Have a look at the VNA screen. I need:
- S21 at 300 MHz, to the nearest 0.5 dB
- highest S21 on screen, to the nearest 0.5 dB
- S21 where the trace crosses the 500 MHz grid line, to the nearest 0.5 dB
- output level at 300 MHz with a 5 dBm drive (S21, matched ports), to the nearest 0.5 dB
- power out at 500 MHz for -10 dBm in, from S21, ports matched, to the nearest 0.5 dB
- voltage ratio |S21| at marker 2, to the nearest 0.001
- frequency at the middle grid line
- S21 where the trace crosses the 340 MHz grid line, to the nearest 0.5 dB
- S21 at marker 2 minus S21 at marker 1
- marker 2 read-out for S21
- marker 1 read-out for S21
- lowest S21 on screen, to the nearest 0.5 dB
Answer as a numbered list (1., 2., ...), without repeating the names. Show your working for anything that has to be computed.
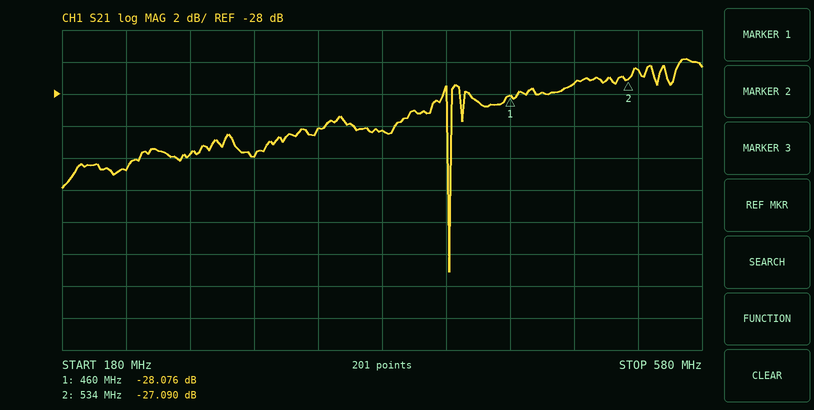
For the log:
1. -32.0 dB
2. -26.0 dB
3. -27.5 dB
4. 5 dBm + (-32.0 dB) = -27.0 dBm
5. -10 dBm + (-27.5 dB) = -37.5 dBm
6. 10^(-27.09/20) ≈ 0.044
7. 380 MHz
8. -30.0 dB
9. -27.09 − (-28.076) = 0.986 dB
10. -27.090 dB
11. -28.076 dB
12. -39.0 dB
